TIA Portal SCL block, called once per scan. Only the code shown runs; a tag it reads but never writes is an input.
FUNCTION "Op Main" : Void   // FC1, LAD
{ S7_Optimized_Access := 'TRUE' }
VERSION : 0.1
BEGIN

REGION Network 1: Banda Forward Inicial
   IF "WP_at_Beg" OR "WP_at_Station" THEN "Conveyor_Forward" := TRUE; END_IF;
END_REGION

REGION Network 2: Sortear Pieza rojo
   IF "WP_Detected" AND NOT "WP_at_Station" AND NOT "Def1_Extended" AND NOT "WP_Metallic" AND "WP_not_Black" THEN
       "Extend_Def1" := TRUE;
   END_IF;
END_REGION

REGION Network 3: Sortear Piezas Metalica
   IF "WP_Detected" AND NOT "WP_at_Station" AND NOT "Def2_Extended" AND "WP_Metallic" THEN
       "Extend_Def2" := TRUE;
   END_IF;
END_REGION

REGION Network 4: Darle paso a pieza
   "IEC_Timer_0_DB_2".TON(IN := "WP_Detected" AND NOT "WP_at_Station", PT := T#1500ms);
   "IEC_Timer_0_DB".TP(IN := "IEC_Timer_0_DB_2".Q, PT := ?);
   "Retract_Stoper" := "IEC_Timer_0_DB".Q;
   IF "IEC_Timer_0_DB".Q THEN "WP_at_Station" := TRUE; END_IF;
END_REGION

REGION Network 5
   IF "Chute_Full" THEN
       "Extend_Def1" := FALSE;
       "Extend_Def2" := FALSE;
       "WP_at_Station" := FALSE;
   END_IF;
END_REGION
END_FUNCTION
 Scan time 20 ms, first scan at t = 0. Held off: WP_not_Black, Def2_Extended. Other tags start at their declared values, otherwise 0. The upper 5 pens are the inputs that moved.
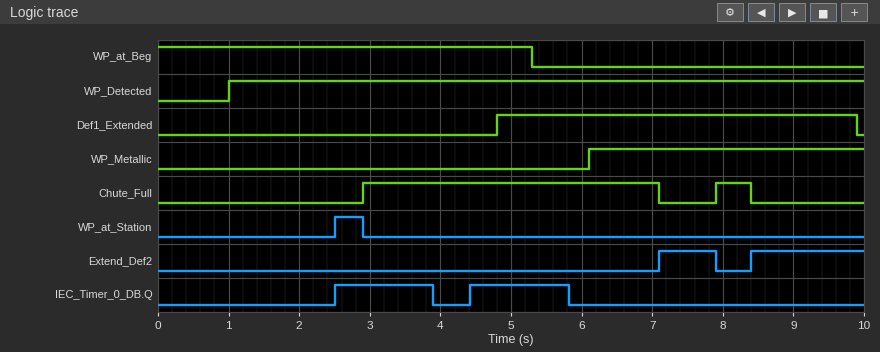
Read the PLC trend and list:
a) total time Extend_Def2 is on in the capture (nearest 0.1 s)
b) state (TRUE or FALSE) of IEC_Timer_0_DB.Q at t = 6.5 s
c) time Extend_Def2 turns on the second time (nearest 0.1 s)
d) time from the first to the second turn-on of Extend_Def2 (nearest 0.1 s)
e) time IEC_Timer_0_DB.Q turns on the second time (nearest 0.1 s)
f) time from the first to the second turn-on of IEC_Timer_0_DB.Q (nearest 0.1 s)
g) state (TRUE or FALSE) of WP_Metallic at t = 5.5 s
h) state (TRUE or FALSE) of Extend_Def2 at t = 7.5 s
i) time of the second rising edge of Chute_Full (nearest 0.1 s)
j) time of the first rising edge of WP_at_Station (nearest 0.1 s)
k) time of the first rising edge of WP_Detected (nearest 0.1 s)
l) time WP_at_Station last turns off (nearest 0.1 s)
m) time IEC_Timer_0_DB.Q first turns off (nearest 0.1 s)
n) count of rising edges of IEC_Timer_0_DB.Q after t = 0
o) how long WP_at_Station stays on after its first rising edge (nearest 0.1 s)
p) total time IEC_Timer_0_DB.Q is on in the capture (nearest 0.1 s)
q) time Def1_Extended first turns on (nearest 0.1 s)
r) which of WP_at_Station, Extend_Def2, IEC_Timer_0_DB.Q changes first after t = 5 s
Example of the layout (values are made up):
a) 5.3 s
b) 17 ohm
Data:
a) 2.4 s
b) FALSE
c) 8.4 s
d) 1.3 s
e) 4.4 s
f) 1.9 s
g) FALSE
h) TRUE
i) 7.9 s
j) 2.5 s
k) 1.0 s
l) 2.9 s
m) 3.9 s
n) 2
o) 0.4 s
p) 2.8 s
q) 4.8 s
r) IEC_Timer_0_DB.Q
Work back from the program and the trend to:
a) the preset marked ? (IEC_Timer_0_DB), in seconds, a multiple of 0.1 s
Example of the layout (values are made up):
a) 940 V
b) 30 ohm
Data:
a) 1.4 s
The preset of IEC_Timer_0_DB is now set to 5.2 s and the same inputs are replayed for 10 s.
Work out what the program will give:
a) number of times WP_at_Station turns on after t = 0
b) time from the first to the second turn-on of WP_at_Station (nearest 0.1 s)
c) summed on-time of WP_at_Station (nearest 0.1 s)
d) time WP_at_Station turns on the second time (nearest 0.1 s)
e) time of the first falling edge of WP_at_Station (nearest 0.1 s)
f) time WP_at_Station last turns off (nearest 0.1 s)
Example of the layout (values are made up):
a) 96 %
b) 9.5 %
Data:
a) 3
b) 4.6 s
c) 1.8 s
d) 7.1 s
e) 2.9 s
f) 7.9 s
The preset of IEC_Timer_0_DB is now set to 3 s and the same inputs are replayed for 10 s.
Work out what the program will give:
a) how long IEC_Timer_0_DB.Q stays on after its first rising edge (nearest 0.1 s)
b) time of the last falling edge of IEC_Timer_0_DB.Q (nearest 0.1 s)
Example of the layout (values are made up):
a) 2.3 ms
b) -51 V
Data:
a) 3.0 s
b) 5.5 s
